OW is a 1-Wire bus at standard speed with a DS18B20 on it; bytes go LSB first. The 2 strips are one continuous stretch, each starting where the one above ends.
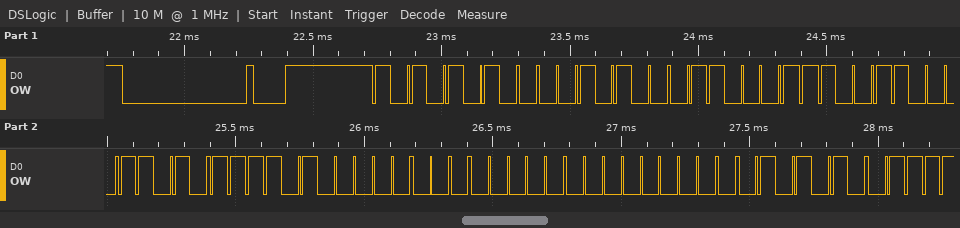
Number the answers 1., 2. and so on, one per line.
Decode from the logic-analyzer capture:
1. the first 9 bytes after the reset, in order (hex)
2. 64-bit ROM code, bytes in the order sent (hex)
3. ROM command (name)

1. 55 28 C6 19 EB 05 00 00 54
2. 28 C6 19 EB 05 00 00 54
3. Match ROM
